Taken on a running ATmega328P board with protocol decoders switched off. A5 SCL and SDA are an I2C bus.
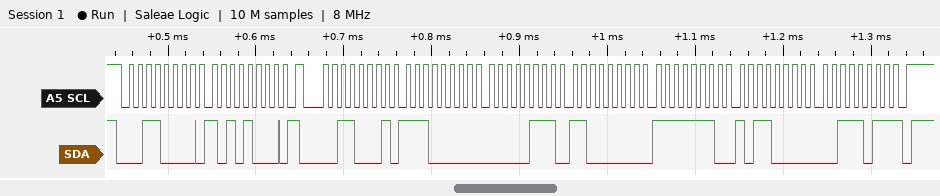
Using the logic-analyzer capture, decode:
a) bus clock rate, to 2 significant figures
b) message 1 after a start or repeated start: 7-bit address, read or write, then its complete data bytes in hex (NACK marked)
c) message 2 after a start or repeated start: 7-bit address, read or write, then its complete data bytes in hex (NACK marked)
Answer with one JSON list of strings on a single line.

["100 kHz", "0x18 write: A8", "0x18 read: E0 07 C0 FE B0 3B NACK"]
